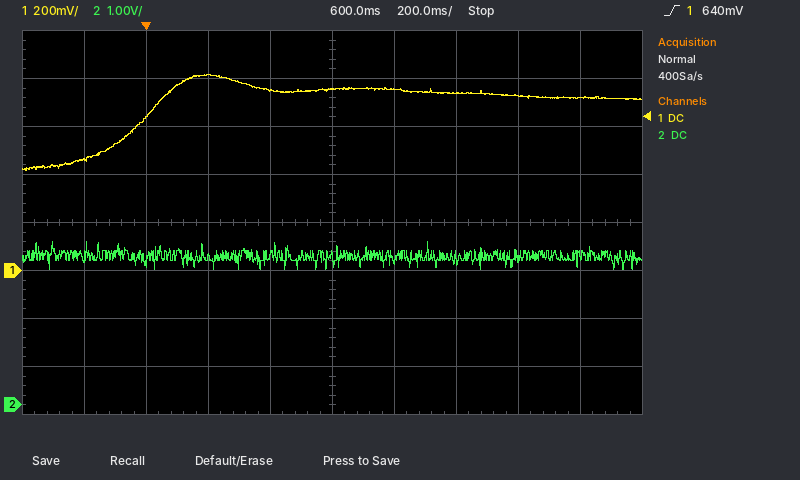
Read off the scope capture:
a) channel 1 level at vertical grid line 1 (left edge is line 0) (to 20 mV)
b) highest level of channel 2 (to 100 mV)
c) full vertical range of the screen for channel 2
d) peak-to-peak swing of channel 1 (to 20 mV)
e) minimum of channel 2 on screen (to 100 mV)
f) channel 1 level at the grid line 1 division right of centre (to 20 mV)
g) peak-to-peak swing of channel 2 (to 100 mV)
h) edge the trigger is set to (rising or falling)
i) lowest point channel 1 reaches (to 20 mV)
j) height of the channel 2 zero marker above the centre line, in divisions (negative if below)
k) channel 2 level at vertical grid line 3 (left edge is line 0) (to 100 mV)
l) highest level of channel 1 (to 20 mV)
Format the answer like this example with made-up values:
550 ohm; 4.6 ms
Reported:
460 mV; 3.4 V; 8 V; 400 mV; 2.8 V; 760 mV; 600 mV; rising; 420 mV; -3.8 div; 3.1 V; 820 mV
